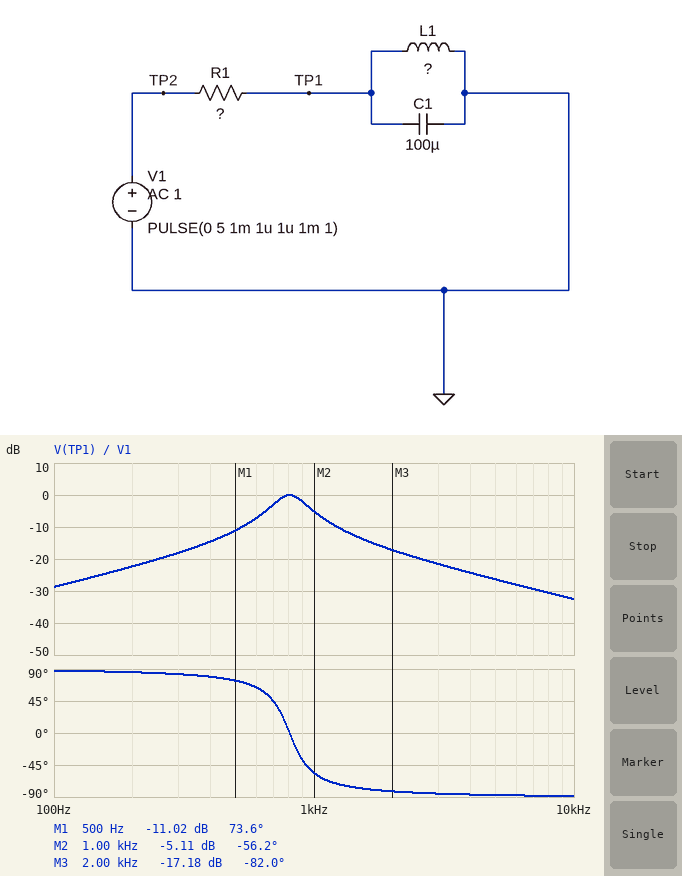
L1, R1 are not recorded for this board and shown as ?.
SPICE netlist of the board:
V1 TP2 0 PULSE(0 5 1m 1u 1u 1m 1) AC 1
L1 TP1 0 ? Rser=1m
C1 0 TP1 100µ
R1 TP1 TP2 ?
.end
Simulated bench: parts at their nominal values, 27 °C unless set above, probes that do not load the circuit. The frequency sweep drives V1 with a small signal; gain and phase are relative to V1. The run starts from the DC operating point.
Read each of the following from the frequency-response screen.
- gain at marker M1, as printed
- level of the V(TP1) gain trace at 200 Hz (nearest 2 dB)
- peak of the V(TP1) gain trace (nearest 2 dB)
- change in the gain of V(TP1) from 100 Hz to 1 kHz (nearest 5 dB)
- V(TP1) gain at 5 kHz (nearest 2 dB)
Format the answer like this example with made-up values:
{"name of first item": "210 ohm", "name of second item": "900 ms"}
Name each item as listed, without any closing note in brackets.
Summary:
{"gain at marker M1, as printed": "-11.02 dB", "level of the V(TP1) gain trace at 200 Hz": "-22 dB", "peak of the V(TP1) gain trace": "0 dB", "change in the gain of V(TP1) from 100 Hz to 1 kHz": "25 dB", "V(TP1) gain at 5 kHz": "-26 dB"}
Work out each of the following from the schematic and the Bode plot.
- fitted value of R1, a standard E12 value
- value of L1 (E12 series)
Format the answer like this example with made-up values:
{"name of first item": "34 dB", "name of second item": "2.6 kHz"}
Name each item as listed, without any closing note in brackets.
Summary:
{"fitted value of R1, a standard E12 value": "6.8 Ω", "value of L1": "390 µH"}
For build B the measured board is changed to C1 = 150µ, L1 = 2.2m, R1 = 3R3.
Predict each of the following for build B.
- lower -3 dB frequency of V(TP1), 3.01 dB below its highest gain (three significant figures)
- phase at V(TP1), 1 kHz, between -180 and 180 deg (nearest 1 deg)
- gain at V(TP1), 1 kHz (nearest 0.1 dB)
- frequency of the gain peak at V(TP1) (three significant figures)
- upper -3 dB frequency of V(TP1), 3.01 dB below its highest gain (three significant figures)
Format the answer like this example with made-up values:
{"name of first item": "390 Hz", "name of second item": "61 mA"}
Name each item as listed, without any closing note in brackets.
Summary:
{"lower -3 dB frequency of V(TP1), 3.01 dB below its highest gain": "160 Hz", "phase at V(TP1), 1 kHz, between -180 and 180 deg": "-71 deg", "gain at V(TP1), 1 kHz": "-9.7 dB", "frequency of the gain peak at V(TP1)": "277 Hz", "upper -3 dB frequency of V(TP1), 3.01 dB below its highest gain": "481 Hz"}
